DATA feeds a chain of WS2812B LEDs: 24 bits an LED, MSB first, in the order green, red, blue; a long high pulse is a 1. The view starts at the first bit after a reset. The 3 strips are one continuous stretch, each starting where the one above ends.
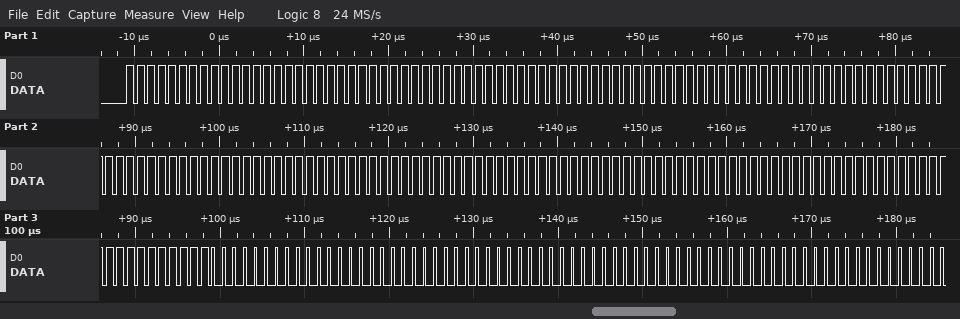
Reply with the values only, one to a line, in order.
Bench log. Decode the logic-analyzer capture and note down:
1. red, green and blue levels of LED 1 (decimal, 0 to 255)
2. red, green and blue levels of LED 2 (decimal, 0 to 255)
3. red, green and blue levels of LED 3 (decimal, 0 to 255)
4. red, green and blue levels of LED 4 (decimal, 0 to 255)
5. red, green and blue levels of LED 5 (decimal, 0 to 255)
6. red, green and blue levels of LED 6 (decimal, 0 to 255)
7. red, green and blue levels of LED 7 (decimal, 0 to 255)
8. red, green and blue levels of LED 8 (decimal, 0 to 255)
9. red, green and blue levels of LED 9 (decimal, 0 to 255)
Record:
255, 255, 255
255, 255, 255
255, 255, 255
255, 255, 255
255, 255, 255
255, 255, 255
255, 255, 255
0, 0, 0
0, 0, 0
